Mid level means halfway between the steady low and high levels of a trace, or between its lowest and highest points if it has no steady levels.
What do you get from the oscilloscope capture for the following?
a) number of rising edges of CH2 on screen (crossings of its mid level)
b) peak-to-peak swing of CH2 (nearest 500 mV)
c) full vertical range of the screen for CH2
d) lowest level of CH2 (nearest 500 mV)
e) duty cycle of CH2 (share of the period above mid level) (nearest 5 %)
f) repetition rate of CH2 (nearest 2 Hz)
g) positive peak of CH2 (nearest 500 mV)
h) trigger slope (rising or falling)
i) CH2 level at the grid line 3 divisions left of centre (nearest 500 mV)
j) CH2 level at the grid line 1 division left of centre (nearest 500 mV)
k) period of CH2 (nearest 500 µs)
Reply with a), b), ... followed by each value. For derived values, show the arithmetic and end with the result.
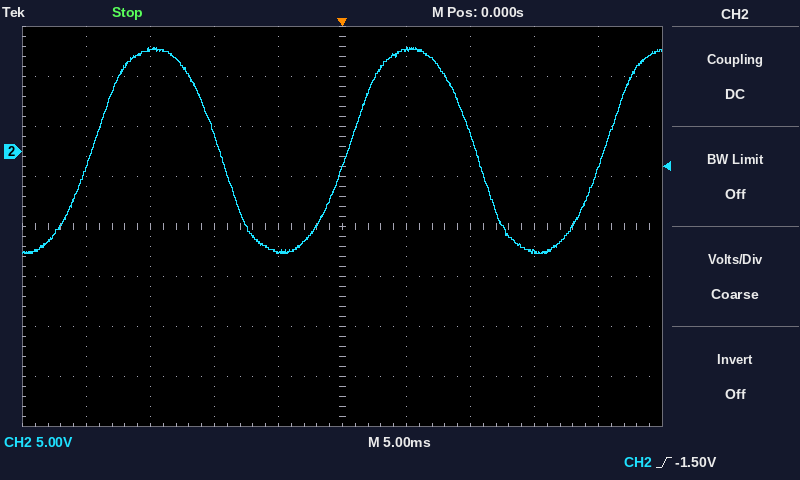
a) 3
b) 10.5 V − (-10.0 V) = 20.5 V
c) 40 V
d) -10.0 V
e) 50 %
f) 1 / 20.0 ms ≈ 50 Hz
g) 10.5 V
h) rising
i) 10.0 V
j) -10.0 V
k) 20.0 ms
